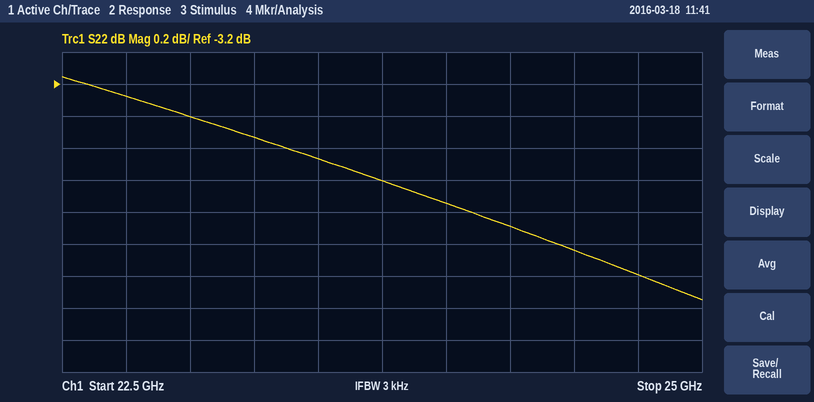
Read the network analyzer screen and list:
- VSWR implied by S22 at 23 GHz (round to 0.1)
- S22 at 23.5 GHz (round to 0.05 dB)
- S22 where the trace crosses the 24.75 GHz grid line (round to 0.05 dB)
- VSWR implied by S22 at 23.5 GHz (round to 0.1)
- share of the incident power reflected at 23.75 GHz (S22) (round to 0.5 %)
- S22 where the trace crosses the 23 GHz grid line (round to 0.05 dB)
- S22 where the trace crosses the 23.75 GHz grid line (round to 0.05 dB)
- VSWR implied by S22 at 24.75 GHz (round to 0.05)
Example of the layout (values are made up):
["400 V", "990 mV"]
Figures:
["5.2", "-3.65 dB", "-4.40 dB", "4.8", "41.5 %", "-3.40 dB", "-3.80 dB", "4.05"]
